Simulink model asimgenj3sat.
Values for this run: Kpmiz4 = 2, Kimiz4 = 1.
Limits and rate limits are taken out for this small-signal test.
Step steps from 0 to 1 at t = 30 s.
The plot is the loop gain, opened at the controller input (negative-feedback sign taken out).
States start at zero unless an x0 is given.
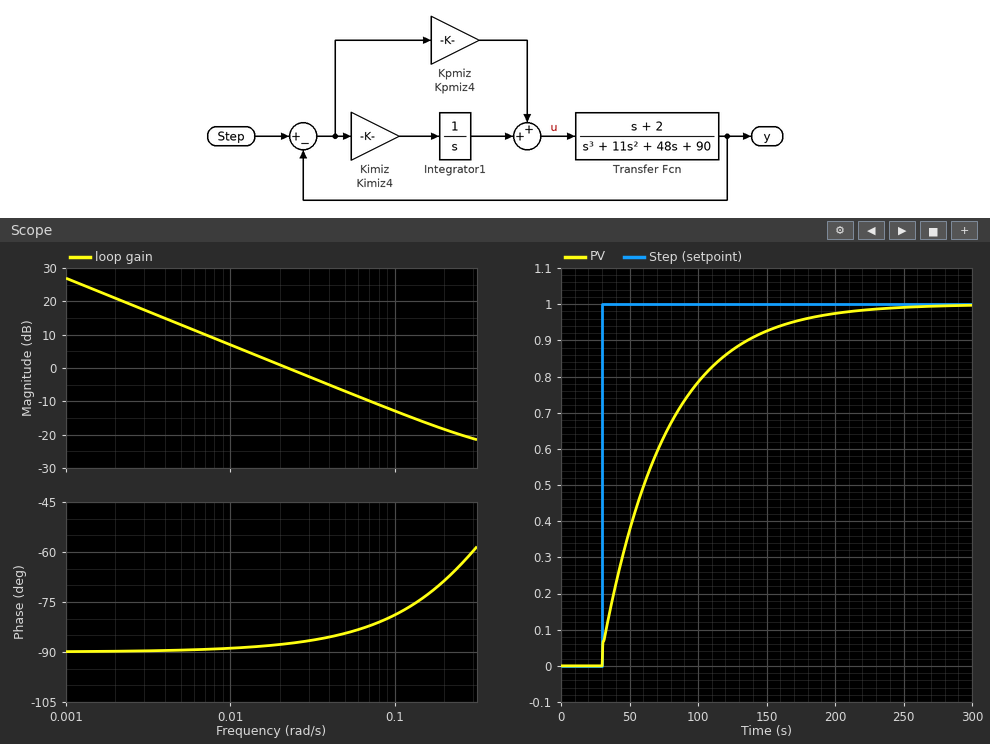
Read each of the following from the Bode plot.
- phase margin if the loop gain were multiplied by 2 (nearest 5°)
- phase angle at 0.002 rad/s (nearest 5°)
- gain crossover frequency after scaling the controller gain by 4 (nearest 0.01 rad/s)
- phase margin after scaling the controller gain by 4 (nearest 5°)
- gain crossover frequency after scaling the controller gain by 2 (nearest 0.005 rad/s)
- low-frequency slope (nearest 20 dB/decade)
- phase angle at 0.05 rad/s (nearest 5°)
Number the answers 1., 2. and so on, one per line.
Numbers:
1. 95°
2. -90°
3. 0.09 rad/s
4. 100°
5. 0.045 rad/s
6. -20 dB/decade
7. -85°
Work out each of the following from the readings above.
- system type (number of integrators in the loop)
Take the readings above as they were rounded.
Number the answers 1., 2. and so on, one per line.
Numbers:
1. 1
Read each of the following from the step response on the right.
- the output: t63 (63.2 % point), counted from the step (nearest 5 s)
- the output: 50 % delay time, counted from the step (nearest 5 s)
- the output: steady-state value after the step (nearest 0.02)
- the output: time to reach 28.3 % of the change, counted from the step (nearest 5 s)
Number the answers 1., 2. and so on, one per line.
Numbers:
1. 45 s
2. 30 s
3. 1.00
4. 15 s
